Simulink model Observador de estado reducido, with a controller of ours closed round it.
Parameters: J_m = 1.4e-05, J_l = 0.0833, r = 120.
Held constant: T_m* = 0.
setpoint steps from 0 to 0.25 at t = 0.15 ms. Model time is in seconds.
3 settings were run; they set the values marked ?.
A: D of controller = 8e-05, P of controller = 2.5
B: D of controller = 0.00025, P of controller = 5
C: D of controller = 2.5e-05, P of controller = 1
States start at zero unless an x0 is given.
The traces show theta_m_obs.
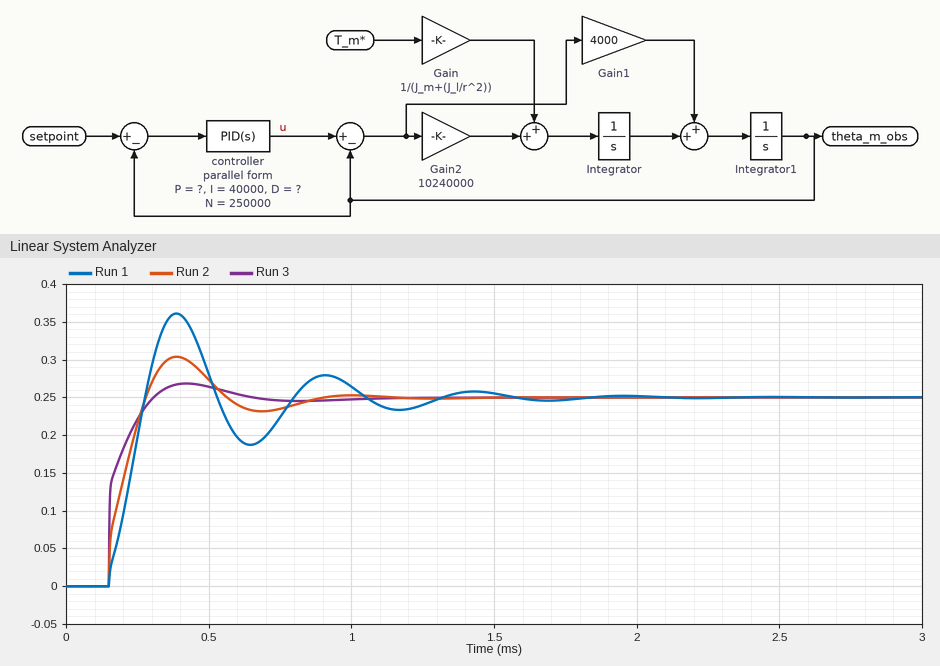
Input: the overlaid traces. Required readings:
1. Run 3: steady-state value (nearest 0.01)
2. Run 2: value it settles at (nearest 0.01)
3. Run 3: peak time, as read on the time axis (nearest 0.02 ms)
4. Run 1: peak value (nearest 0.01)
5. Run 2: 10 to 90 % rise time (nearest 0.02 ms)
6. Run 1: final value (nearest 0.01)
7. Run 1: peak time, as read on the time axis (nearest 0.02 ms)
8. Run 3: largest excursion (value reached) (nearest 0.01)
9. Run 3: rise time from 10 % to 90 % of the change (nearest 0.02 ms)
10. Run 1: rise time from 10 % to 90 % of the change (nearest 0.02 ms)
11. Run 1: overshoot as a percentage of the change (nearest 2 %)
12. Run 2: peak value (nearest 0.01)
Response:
0.25
0.25
0.42 ms
0.36
0.10 ms
0.25
0.38 ms
0.27
0.10 ms
0.10 ms
44 %
0.30
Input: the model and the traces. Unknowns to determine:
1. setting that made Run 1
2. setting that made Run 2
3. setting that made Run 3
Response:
C
A
B
